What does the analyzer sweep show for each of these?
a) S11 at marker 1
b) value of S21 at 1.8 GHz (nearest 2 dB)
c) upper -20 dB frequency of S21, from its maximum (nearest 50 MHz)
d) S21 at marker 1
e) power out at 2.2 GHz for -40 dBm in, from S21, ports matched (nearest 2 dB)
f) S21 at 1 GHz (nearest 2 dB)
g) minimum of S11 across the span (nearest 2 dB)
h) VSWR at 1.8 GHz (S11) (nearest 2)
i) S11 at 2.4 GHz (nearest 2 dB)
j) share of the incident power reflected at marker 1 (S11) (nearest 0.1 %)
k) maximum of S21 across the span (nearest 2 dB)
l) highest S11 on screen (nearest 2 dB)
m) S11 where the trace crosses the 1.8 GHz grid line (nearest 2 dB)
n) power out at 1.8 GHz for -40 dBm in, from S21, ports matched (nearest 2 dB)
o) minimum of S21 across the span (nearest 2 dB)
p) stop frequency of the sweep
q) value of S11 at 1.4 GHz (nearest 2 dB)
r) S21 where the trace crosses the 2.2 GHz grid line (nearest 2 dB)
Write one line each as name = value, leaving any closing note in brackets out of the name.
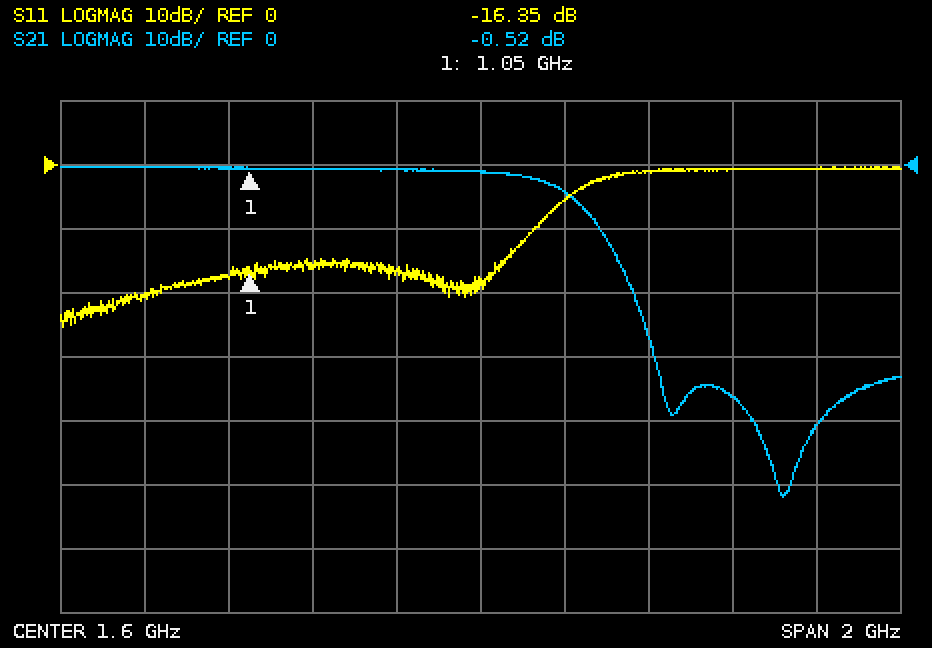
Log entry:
S11 at marker 1 = -16.35 dB
value of S21 at 1.8 GHz = -4 dB
upper -20 dB frequency of S21, from its maximum = 1.95 GHz
S21 at marker 1 = -0.52 dB
power out at 2.2 GHz for -40 dBm in, from S21, ports matched = -76 dBm
S21 at 1 GHz = 0 dB
minimum of S11 across the span = -26 dB
VSWR at 1.8 GHz (S11) = 4
S11 at 2.4 GHz = 0 dB
share of the incident power reflected at marker 1 (S11) = 2.3 %
maximum of S21 across the span = 0 dB
highest S11 on screen = 0 dB
S11 where the trace crosses the 1.8 GHz grid line = -6 dB
power out at 1.8 GHz for -40 dBm in, from S21, ports matched = -44 dBm
minimum of S21 across the span = -52 dB
stop frequency of the sweep = 2.6 GHz
value of S11 at 1.4 GHz = -16 dB
S21 where the trace crosses the 2.2 GHz grid line = -36 dB
